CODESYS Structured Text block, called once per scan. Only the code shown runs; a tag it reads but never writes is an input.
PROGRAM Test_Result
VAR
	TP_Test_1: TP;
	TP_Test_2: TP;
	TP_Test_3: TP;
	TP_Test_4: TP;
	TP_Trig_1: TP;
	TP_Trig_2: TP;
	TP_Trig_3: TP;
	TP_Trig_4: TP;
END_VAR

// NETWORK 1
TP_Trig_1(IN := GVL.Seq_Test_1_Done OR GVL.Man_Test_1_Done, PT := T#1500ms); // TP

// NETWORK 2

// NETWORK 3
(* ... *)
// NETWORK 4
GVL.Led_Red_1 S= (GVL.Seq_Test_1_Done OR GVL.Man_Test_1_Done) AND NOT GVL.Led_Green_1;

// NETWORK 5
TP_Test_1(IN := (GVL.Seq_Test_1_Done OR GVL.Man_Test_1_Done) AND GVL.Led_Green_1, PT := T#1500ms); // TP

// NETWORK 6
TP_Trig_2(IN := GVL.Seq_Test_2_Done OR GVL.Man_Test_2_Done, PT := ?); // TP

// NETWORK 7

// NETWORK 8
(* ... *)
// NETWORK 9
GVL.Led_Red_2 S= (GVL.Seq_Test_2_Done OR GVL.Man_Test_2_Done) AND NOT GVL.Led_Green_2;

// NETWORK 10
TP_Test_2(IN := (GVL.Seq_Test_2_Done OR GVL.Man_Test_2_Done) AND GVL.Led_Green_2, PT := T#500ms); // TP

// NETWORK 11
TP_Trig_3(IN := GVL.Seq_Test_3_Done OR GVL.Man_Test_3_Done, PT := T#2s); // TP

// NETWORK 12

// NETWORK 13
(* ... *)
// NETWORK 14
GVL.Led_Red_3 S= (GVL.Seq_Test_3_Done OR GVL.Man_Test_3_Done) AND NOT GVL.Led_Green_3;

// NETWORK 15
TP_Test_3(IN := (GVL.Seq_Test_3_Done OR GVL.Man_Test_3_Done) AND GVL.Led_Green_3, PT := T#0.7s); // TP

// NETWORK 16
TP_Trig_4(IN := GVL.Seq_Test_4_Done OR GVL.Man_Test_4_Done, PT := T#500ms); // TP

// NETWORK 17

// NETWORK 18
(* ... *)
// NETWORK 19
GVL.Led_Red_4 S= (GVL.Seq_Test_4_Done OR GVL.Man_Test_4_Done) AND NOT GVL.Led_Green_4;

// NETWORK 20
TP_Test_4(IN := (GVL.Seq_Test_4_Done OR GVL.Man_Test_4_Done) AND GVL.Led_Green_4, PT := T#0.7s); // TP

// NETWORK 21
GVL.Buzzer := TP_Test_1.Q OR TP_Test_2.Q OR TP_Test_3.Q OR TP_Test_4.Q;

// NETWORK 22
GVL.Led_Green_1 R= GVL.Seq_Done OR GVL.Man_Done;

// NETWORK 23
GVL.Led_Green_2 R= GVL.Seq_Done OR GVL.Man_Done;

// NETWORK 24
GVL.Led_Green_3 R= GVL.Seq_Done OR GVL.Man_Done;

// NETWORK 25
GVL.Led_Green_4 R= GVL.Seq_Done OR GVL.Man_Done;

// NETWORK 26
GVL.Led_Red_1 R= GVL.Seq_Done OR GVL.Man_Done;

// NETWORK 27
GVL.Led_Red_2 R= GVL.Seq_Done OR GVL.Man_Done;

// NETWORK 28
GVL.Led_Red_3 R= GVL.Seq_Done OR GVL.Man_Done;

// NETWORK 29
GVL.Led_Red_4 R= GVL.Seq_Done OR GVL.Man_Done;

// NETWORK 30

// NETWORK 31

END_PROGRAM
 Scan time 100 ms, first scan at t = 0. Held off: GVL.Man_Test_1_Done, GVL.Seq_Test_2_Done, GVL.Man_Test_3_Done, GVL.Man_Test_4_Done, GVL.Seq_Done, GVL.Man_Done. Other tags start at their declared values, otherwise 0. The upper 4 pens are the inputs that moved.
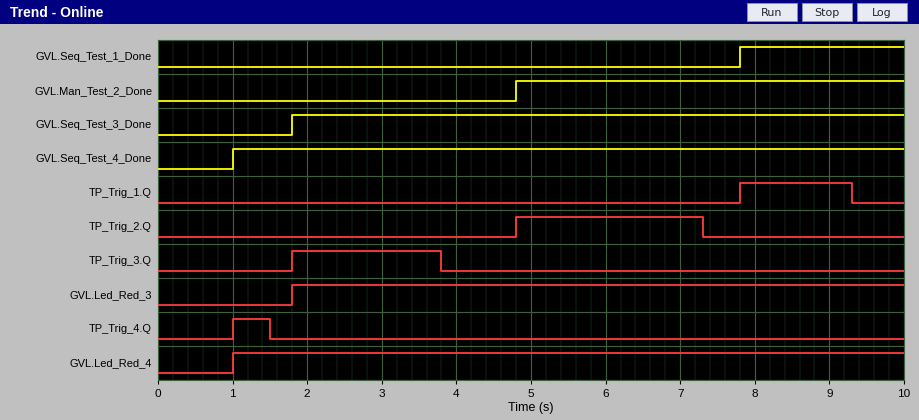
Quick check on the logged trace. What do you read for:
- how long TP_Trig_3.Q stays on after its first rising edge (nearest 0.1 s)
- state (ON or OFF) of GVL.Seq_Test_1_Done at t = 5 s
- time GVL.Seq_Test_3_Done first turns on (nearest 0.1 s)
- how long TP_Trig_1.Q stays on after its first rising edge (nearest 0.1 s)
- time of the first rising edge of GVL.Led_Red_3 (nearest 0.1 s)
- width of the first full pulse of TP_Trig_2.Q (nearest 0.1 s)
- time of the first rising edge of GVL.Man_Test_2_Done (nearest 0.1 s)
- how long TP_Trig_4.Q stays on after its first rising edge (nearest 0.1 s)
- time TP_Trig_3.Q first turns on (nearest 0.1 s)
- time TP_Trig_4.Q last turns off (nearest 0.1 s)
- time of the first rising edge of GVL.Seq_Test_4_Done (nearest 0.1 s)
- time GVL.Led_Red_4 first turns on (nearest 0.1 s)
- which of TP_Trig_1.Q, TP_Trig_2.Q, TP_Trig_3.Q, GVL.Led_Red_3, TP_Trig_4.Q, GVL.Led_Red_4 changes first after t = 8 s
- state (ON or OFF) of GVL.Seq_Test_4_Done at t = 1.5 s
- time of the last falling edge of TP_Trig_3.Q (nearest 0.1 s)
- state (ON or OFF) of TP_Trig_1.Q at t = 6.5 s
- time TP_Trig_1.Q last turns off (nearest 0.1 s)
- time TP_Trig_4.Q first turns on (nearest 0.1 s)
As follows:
2.0 s
OFF
1.8 s
1.5 s
1.8 s
2.5 s
4.8 s
0.5 s
1.8 s
1.5 s
1.0 s
1.0 s
TP_Trig_1.Q
ON
3.8 s
OFF
9.3 s
1.0 s
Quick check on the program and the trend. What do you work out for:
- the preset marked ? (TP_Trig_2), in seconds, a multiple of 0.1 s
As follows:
2.5 s
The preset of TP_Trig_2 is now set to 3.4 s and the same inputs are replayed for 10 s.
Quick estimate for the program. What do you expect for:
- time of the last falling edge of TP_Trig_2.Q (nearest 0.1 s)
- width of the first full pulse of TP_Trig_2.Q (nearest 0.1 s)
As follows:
8.2 s
3.4 s
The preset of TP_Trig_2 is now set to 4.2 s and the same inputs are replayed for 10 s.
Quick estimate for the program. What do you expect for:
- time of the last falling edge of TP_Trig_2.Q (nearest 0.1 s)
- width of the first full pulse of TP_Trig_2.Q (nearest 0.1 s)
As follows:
9.0 s
4.2 s
